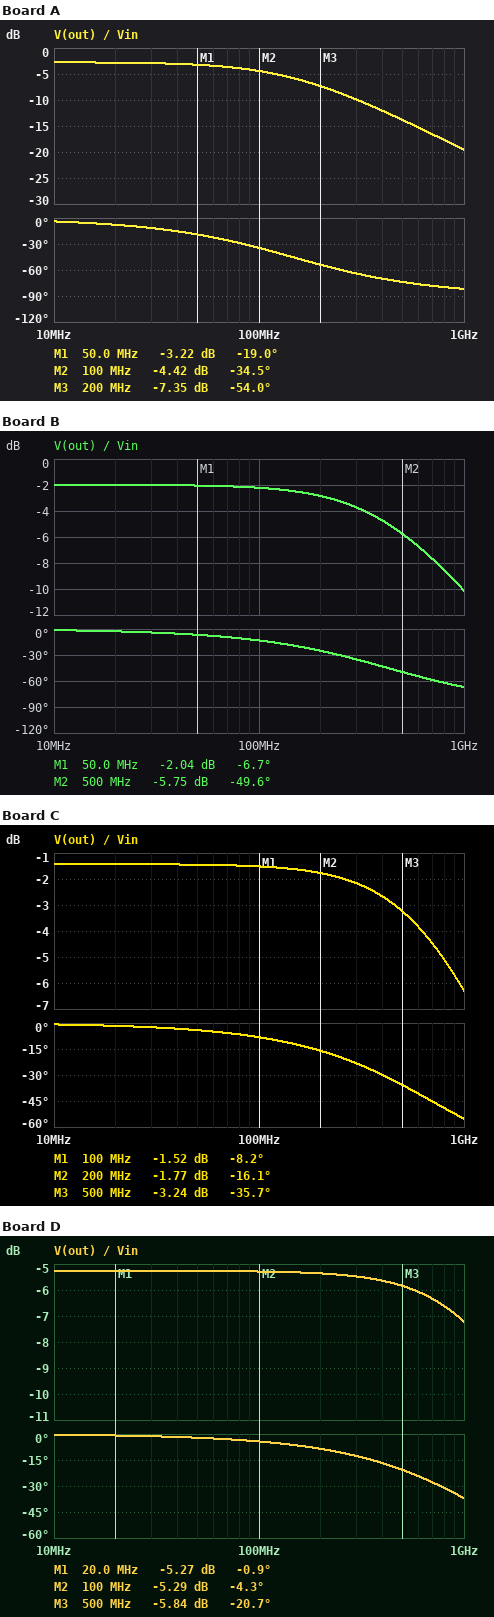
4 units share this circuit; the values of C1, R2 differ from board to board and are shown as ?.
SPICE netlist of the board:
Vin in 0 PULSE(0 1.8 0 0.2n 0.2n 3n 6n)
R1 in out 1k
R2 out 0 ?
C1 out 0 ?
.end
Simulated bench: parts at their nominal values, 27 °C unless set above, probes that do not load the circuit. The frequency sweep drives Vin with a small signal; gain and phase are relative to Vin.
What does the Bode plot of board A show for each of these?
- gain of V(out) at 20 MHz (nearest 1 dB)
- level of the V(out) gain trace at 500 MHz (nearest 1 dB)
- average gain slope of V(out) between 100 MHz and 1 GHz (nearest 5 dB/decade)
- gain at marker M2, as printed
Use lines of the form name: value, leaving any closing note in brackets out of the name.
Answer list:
gain of V(out) at 20 MHz: -3 dB
level of the V(out) gain trace at 500 MHz: -14 dB
average gain slope of V(out) between 100 MHz and 1 GHz: -15 dB/decade
gain at marker M2, as printed: -4.42 dB
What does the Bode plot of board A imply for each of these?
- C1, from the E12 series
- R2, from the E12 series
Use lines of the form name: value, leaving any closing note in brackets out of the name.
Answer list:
C1, from the E12 series: 1.5 pF
R2, from the E12 series: 2.7 kΩ
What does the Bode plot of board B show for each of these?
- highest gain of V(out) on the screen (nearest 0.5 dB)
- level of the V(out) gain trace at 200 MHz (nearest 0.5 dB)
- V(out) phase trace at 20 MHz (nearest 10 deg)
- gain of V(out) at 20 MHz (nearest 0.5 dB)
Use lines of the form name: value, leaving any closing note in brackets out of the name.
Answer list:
highest gain of V(out) on the screen: -2.0 dB
level of the V(out) gain trace at 200 MHz: -3.0 dB
V(out) phase trace at 20 MHz: 0 deg
gain of V(out) at 20 MHz: -2.0 dB
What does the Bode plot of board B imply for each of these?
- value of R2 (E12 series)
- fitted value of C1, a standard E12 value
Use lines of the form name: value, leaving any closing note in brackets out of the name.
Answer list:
value of R2: 3.9 kΩ
fitted value of C1, a standard E12 value: 470 fF
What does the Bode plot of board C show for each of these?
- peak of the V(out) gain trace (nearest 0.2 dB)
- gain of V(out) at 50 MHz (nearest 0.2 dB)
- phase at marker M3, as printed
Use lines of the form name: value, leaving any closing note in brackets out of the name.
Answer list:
peak of the V(out) gain trace: -1.4 dB
gain of V(out) at 50 MHz: -1.4 dB
phase at marker M3, as printed: -35.7 deg
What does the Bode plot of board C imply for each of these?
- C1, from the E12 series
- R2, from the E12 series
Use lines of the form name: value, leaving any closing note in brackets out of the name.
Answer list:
C1, from the E12 series: 270 fF
R2, from the E12 series: 5.6 kΩ
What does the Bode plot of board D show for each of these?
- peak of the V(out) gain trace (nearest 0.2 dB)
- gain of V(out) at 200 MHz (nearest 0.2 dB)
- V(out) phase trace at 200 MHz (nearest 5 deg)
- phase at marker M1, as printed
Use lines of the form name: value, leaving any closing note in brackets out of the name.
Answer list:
peak of the V(out) gain trace: -5.2 dB
gain of V(out) at 200 MHz: -5.4 dB
V(out) phase trace at 200 MHz: -10 deg
phase at marker M1, as printed: -0.9 deg
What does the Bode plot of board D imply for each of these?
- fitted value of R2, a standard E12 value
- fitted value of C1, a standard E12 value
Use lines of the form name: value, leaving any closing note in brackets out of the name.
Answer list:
fitted value of R2, a standard E12 value: 1.2 kΩ
fitted value of C1, a standard E12 value: 220 fF
